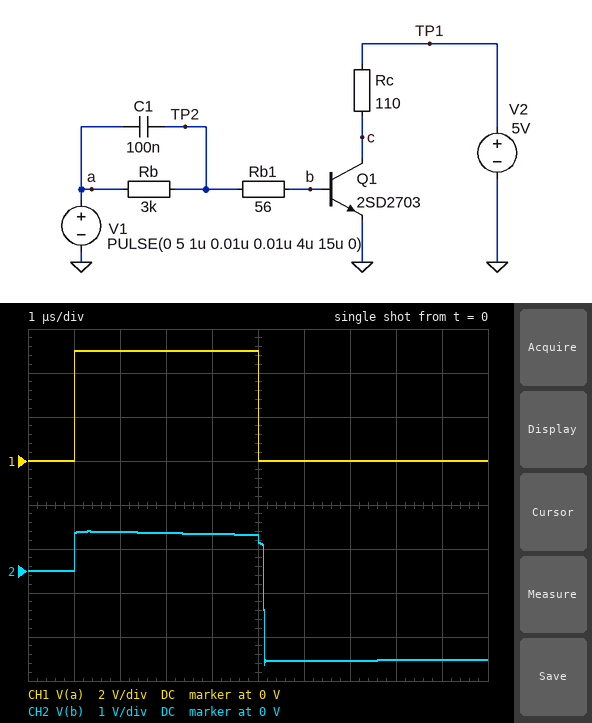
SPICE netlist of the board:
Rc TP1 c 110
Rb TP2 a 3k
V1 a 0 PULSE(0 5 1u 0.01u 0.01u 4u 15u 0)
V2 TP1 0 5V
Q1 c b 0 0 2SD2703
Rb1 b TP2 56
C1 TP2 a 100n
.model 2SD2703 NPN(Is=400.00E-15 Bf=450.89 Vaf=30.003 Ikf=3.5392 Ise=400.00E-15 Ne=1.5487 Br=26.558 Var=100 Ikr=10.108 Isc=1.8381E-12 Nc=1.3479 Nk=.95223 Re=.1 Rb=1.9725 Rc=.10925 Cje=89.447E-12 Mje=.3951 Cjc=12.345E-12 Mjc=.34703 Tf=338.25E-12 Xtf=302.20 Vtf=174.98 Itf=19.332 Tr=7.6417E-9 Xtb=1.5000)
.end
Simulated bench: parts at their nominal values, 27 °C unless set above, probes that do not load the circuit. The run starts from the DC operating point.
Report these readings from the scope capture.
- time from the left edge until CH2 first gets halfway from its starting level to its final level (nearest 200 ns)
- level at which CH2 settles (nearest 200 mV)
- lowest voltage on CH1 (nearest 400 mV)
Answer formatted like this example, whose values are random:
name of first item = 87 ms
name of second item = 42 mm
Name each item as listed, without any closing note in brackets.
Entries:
time from the left edge until CH2 first gets halfway from its starting level to its final level = 5.2 µs
level at which CH2 settles = -2.0 V
lowest voltage on CH1 = 0 V
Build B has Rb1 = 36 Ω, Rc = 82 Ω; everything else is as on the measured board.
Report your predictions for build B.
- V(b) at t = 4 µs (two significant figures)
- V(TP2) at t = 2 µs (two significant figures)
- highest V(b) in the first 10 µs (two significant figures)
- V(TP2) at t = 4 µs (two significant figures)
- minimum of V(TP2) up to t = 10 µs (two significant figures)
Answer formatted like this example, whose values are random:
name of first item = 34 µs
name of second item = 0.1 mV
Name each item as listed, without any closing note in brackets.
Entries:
V(b) at t = 4 µs = 860 mV
V(TP2) at t = 2 µs = 4.0 V
highest V(b) in the first 10 µs = 980 mV
V(TP2) at t = 4 µs = 2.7 V
minimum of V(TP2) up to t = 10 µs = -2.7 V
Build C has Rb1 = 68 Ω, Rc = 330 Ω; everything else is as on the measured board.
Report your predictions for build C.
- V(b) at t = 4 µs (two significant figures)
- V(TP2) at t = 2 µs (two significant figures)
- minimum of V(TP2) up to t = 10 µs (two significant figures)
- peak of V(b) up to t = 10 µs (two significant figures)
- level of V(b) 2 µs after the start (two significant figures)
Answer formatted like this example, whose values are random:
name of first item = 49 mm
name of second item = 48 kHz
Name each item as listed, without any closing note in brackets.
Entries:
V(b) at t = 4 µs = 820 mV
V(TP2) at t = 2 µs = 4.4 V
minimum of V(TP2) up to t = 10 µs = -1.8 V
peak of V(b) up to t = 10 µs = 870 mV
level of V(b) 2 µs after the start = 860 mV
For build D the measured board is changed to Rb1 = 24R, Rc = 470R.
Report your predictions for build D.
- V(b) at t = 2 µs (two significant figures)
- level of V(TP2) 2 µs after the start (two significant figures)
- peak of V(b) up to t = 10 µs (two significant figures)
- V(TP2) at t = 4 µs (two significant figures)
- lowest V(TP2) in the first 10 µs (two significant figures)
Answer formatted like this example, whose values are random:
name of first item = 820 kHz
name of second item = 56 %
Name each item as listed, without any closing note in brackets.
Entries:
V(b) at t = 2 µs = 1.0 V
level of V(TP2) 2 µs after the start = 3.7 V
peak of V(b) up to t = 10 µs = 1.1 V
V(TP2) at t = 4 µs = 2.1 V
lowest V(TP2) in the first 10 µs = -3.3 V
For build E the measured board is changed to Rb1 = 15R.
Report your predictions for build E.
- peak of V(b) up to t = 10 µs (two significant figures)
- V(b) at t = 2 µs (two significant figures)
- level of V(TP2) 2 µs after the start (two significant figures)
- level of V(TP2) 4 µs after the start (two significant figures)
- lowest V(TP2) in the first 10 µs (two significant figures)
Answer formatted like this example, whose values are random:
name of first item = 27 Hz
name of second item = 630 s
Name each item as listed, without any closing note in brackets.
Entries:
peak of V(b) up to t = 10 µs = 1.3 V
V(b) at t = 2 µs = 1.1 V
level of V(TP2) 2 µs after the start = 3.1 V
level of V(TP2) 4 µs after the start = 1.5 V
lowest V(TP2) in the first 10 µs = -3.8 V
